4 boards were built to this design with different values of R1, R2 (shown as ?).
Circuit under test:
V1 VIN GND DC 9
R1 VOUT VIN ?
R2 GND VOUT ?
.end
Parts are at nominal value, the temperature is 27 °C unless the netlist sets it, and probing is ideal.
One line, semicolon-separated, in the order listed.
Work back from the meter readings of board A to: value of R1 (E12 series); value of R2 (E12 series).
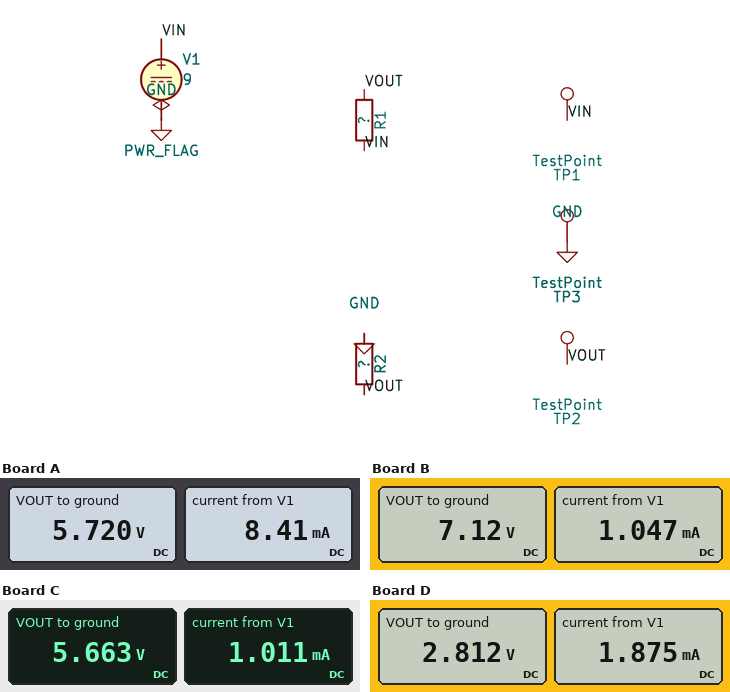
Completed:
390 Ω; 680 Ω
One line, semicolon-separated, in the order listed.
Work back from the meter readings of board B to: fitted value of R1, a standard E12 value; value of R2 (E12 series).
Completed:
1.8 kΩ; 6.8 kΩ
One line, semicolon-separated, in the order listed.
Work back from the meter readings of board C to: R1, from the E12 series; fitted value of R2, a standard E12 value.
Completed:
3.3 kΩ; 5.6 kΩ
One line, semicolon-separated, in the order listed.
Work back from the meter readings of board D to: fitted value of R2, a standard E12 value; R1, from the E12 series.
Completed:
1.5 kΩ; 3.3 kΩ
